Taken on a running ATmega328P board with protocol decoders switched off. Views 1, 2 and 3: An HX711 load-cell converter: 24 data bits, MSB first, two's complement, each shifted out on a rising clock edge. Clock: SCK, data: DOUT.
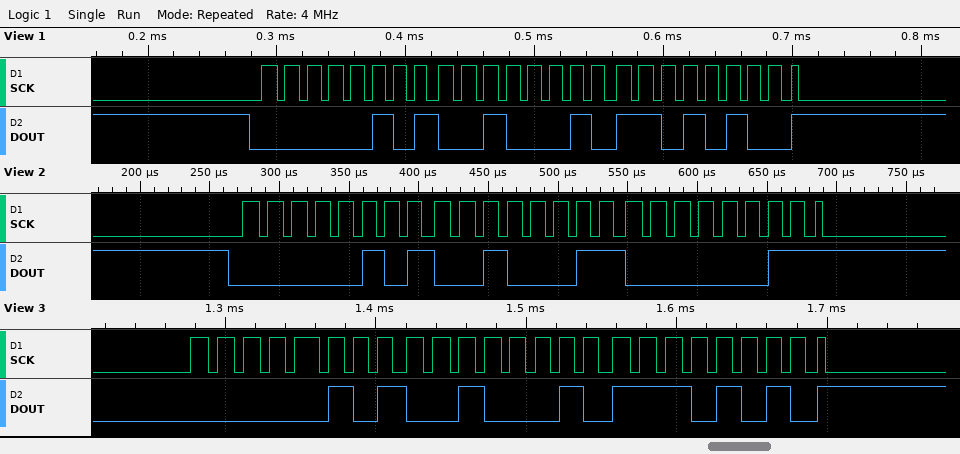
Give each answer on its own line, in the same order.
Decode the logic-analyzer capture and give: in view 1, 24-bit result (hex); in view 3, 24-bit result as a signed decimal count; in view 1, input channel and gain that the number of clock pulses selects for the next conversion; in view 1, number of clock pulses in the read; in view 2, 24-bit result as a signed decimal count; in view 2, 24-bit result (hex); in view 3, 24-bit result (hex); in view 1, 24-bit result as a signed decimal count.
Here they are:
0x0522D4
336618
channel A, gain 128
25
336643
0x052303
0x0522EA
336596
